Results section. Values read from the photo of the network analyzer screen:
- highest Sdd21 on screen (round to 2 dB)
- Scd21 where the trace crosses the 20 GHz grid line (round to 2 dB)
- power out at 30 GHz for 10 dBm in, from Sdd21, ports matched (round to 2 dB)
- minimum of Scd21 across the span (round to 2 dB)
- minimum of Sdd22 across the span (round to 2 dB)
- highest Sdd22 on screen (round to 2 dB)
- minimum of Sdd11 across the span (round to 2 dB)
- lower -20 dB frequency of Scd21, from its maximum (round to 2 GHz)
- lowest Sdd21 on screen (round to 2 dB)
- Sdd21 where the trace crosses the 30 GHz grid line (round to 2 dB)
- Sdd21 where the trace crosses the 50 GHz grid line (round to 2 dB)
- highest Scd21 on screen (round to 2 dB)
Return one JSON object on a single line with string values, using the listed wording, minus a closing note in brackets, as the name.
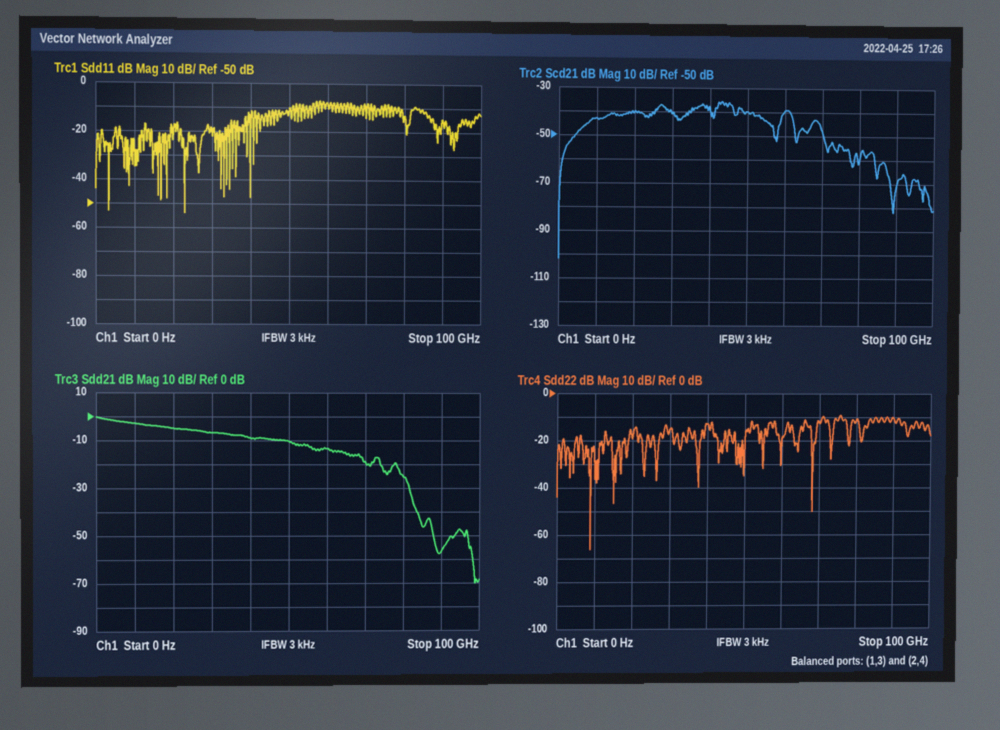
{"highest Sdd21 on screen": "0 dB", "Scd21 where the trace crosses the 20 GHz grid line": "-40 dB", "power out at 30 GHz for 10 dBm in, from Sdd21, ports matched": "4 dBm", "minimum of Scd21 across the span": "-102 dB", "minimum of Sdd22 across the span": "-66 dB", "highest Sdd22 on screen": "-10 dB", "minimum of Sdd11 across the span": "-54 dB", "lower -20 dB frequency of Scd21, from its maximum": "2 GHz", "lowest Sdd21 on screen": "-70 dB", "Sdd21 where the trace crosses the 30 GHz grid line": "-6 dB", "Sdd21 where the trace crosses the 50 GHz grid line": "-10 dB", "highest Scd21 on screen": "-36 dB"}
